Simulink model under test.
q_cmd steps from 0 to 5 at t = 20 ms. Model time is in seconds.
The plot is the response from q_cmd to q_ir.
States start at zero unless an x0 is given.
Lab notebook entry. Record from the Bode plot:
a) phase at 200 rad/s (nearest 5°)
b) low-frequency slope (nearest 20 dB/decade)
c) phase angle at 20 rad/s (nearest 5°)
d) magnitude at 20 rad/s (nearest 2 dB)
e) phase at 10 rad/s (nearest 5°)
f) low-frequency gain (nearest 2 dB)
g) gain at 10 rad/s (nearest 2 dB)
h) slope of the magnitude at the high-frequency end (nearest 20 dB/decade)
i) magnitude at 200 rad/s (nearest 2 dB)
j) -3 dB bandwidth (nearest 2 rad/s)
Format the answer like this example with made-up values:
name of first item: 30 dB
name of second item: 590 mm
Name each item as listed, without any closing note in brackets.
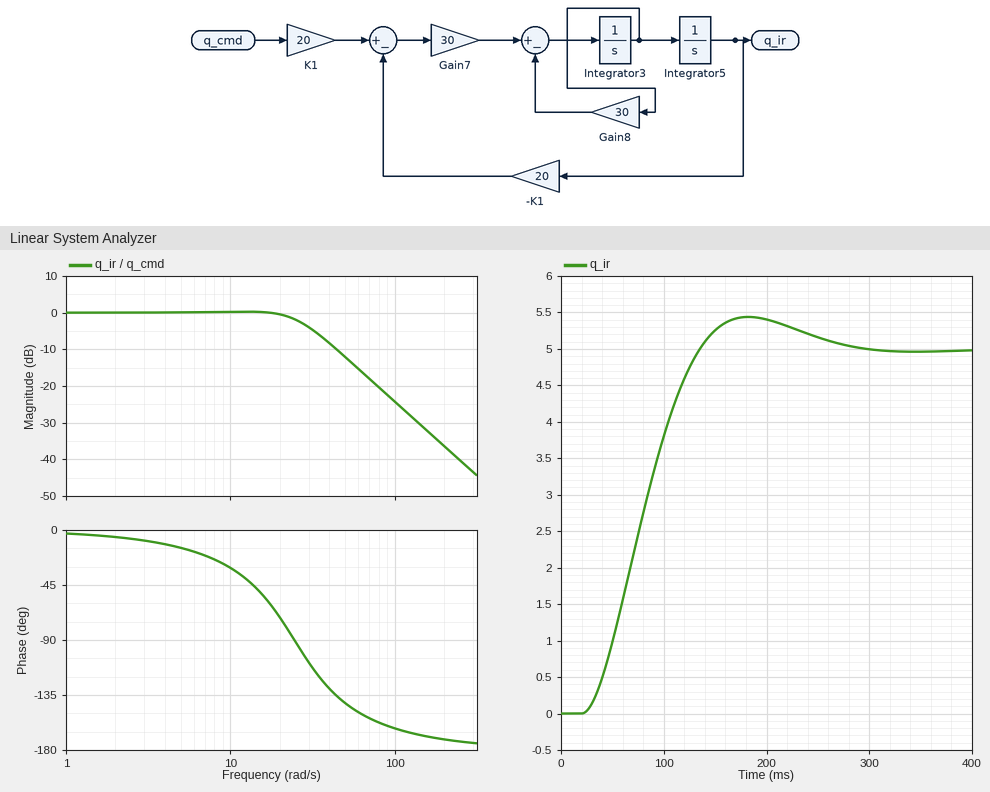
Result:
phase at 200 rad/s: -170°
low-frequency slope: 0 dB/decade
phase angle at 20 rad/s: -70°
magnitude at 20 rad/s: 0 dB
phase at 10 rad/s: -30°
low-frequency gain: 0 dB
gain at 10 rad/s: 0 dB
slope of the magnitude at the high-frequency end: -40 dB/decade
magnitude at 200 rad/s: -36 dB
-3 dB bandwidth: 28 rad/s
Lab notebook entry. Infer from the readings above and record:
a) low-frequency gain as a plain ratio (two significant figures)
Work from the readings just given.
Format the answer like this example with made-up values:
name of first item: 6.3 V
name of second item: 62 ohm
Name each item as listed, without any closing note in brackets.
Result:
low-frequency gain as a plain ratio: 1.0
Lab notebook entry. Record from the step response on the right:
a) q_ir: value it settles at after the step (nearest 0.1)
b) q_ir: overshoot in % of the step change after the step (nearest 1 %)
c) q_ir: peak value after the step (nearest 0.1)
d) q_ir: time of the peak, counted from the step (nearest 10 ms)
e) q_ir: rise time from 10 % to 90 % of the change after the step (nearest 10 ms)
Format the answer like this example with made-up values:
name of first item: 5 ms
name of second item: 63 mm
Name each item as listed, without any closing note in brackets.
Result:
q_ir: value it settles at after the step: 5.0
q_ir: overshoot in % of the step change after the step: 9 %
q_ir: peak value after the step: 5.4
q_ir: time of the peak, counted from the step: 160 ms
q_ir: rise time from 10 % to 90 % of the change after the step: 80 ms
